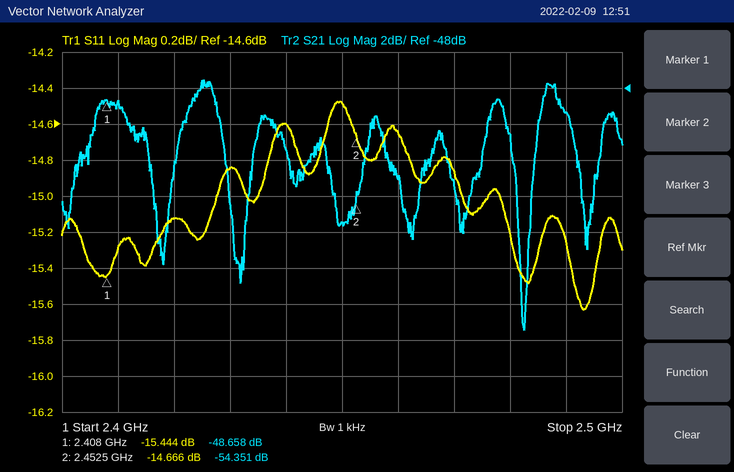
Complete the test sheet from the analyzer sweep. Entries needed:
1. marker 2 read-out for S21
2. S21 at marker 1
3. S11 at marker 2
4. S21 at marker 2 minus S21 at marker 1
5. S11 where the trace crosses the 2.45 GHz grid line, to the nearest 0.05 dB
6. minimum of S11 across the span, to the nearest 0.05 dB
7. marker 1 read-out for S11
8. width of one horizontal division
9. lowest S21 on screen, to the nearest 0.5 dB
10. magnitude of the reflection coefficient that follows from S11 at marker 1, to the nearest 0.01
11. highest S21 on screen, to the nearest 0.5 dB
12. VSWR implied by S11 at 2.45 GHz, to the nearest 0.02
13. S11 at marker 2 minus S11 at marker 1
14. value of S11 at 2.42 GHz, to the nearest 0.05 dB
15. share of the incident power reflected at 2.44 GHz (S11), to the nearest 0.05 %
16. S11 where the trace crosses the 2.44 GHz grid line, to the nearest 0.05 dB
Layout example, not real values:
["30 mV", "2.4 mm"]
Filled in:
["-54.351 dB", "-48.658 dB", "-14.666 dB", "-5.693 dB", "-14.50 dB", "-15.65 dB", "-15.444 dB", "10 MHz", "-61.5 dB", "0.17", "-47.5 dB", "1.46", "0.778 dB", "-15.10 dB", "3.45 %", "-14.60 dB"]
